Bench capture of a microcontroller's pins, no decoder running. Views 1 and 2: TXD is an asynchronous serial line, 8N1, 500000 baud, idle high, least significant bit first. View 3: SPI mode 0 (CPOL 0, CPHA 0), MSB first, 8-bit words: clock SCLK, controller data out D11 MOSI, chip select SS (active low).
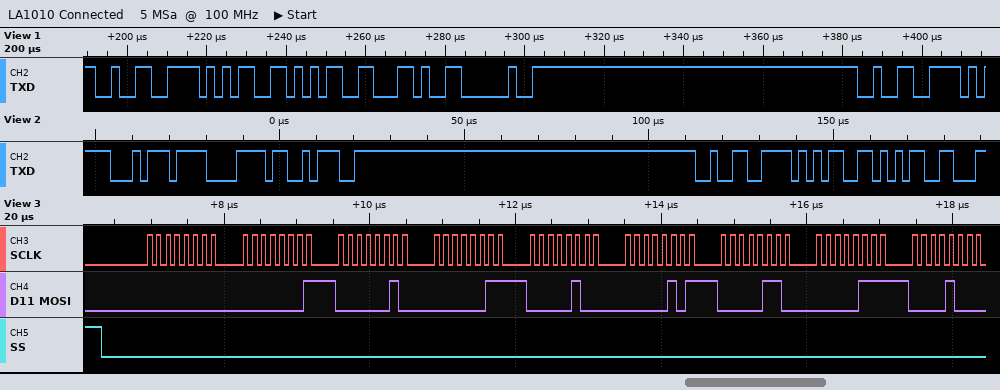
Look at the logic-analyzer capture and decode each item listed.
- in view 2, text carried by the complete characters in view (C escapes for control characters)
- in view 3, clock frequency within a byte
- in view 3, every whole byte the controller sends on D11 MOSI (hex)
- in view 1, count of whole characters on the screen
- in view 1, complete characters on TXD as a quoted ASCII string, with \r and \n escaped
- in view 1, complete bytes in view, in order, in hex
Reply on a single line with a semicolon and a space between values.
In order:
"tx:255"; 8 MHz; 00 01 02 03 04 05 06 07 08; 6; "255, 2"; 32 35 35 2C 20 32
